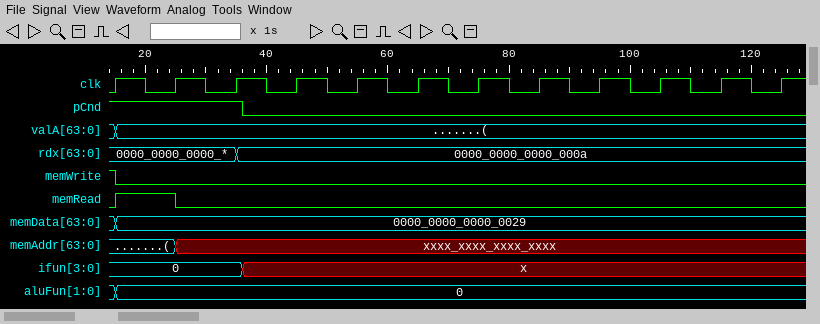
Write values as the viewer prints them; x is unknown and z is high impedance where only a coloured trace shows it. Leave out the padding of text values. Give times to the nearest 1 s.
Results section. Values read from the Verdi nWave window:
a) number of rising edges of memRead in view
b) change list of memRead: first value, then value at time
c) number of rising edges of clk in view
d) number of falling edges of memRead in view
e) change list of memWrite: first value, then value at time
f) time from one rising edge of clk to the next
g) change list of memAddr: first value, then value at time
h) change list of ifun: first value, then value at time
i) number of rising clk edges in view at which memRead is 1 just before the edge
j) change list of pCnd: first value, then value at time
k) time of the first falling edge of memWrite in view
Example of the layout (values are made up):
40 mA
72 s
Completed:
1
0, 1 at 15 s, 0 at 25 s
12
1
1, 0 at 15 s
10 s
(, xxxx_xxxx_xxxx_xxxx at 25 s
0, x at 36 s
1
1, 0 at 36 s
15 s
